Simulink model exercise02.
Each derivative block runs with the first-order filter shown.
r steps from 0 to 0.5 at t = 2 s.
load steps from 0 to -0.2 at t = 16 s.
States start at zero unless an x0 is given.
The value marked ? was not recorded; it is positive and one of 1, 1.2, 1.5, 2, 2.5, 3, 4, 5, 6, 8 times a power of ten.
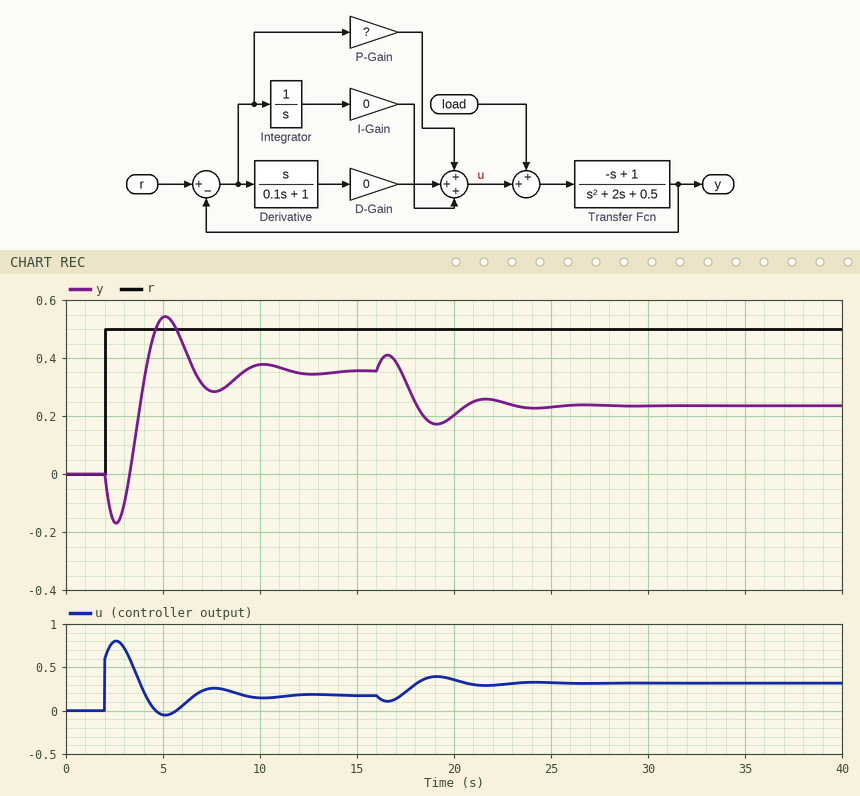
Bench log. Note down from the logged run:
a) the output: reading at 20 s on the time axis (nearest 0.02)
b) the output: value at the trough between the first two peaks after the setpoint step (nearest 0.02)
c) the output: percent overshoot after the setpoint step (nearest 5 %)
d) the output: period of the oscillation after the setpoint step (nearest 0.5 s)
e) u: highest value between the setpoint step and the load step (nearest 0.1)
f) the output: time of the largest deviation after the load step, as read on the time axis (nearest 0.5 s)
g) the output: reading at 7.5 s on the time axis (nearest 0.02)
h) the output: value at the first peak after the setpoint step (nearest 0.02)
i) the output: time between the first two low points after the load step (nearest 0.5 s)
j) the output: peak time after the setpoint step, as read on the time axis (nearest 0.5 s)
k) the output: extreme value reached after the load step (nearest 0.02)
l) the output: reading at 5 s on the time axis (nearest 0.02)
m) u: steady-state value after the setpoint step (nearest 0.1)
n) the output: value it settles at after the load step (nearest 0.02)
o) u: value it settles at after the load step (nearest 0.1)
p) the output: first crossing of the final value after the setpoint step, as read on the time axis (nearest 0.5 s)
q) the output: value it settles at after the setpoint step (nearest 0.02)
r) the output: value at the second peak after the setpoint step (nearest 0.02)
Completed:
0.20
0.28
55 %
5.0 s
0.8
19.0 s
0.28
0.54
5.0 s
5.0 s
0.18
0.54
0.2
0.24
0.3
4.0 s
0.36
0.38
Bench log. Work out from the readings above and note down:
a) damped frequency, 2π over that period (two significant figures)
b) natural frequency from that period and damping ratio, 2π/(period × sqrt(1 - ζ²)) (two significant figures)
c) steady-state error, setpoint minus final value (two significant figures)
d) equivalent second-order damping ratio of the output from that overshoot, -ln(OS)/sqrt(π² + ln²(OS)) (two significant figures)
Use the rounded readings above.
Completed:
1.3 rad/s
1.3 rad/s
0.14
0.19
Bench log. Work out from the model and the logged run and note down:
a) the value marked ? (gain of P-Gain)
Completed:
1.2
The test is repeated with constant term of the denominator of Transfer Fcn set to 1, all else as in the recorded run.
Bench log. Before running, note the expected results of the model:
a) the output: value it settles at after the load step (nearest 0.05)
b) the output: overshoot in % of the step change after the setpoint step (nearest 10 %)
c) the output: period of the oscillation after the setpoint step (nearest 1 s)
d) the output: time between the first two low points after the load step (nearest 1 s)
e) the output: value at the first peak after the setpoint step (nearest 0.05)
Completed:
0.20
70 %
4 s
4 s
0.45
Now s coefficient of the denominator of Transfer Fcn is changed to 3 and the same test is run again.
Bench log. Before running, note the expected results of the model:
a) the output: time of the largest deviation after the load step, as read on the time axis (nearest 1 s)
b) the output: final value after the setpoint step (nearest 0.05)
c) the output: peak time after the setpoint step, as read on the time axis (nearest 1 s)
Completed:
20 s
0.35
6 s
